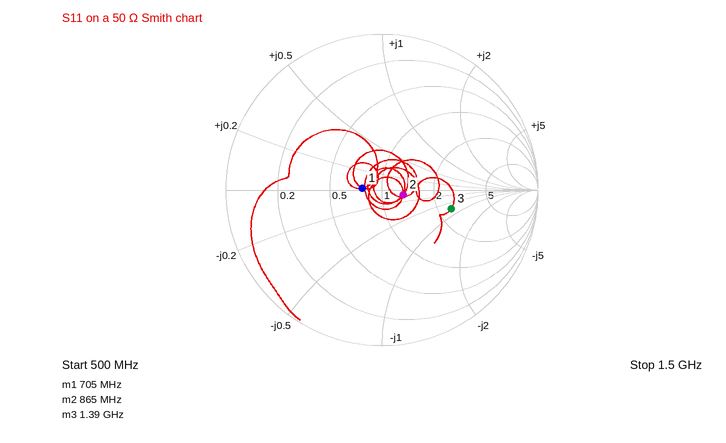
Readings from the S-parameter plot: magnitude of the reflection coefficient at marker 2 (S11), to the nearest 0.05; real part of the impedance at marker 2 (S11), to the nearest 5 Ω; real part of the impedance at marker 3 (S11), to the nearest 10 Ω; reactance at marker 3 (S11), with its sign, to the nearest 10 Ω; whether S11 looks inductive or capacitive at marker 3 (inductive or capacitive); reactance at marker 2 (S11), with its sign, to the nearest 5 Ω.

0.15
65 Ω
120 Ω
-40 Ω
capacitive
-5 Ω
